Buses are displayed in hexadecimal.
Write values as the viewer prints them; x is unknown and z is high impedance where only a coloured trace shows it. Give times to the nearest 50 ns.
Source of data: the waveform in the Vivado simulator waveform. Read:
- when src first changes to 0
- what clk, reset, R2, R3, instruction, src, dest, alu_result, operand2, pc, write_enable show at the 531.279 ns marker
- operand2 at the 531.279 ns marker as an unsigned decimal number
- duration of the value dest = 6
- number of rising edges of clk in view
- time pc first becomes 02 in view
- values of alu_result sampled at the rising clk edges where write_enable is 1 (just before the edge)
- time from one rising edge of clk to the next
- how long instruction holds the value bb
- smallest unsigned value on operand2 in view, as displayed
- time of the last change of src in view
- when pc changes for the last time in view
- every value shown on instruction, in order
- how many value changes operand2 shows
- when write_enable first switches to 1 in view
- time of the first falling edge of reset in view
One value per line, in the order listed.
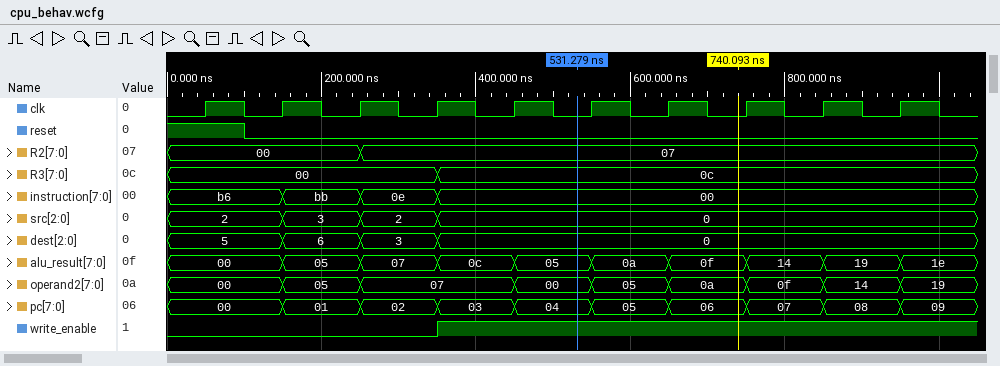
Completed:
350 ns
clk=0, reset=0, R2=07, R3=0c, instruction=00, src=0, dest=0, alu_result=05, operand2=00, pc=04, write_enable=1
0
100 ns
10
250 ns
0c, 05, 0a, 0f, 14, 19
100 ns
100 ns
00
350 ns
950 ns
b6, bb, 0e, 00
8
350 ns
100 ns
